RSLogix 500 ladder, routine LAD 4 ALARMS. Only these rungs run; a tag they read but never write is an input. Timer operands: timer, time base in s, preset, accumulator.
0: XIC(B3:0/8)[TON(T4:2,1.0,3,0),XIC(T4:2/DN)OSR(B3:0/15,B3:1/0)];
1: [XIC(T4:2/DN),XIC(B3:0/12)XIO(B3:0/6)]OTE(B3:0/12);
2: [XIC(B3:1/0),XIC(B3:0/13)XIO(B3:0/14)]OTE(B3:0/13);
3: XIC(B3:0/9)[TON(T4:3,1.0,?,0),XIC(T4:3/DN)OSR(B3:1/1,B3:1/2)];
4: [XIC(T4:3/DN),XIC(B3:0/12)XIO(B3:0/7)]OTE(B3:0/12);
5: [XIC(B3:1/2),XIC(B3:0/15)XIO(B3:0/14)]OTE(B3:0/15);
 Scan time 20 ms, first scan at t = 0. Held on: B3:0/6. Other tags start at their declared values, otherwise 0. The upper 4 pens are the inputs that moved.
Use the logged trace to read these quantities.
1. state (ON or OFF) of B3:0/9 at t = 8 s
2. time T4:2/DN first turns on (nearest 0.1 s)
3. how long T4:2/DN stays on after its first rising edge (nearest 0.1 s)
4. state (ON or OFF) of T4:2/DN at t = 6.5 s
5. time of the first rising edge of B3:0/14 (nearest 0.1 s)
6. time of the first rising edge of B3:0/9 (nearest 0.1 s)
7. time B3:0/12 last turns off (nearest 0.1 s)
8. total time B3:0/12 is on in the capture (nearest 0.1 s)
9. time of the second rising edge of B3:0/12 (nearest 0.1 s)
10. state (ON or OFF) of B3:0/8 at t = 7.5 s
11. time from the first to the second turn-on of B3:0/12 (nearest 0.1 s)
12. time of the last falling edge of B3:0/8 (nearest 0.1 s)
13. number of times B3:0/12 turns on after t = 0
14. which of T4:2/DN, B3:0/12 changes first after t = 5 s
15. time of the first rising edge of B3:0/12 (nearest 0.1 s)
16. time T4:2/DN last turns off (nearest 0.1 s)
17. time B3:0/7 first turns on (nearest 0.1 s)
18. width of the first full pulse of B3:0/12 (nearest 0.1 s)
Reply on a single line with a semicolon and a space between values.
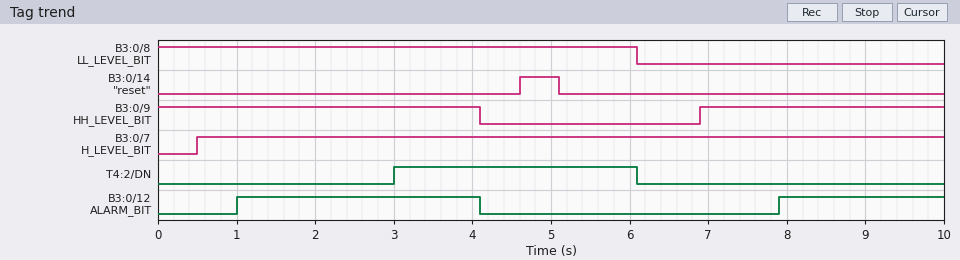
ON; 3.0 s; 3.1 s; OFF; 4.6 s; 6.9 s; 4.1 s; 5.2 s; 7.9 s; OFF; 6.9 s; 6.1 s; 2; T4:2/DN; 1.0 s; 6.1 s; 0.5 s; 3.1 s
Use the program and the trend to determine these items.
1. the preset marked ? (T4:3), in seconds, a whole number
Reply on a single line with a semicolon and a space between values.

1 s
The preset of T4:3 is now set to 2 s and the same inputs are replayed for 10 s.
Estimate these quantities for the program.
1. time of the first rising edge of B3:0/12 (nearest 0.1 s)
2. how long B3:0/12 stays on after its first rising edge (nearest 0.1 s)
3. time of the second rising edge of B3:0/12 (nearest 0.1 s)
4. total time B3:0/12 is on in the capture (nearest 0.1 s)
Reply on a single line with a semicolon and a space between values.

2.0 s; 2.1 s; 8.9 s; 3.2 s
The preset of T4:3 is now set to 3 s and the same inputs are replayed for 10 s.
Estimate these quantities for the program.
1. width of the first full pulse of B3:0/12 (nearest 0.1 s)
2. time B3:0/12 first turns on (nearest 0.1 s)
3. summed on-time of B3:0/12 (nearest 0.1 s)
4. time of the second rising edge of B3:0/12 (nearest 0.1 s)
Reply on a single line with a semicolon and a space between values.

1.1 s; 3.0 s; 1.2 s; 9.9 s
